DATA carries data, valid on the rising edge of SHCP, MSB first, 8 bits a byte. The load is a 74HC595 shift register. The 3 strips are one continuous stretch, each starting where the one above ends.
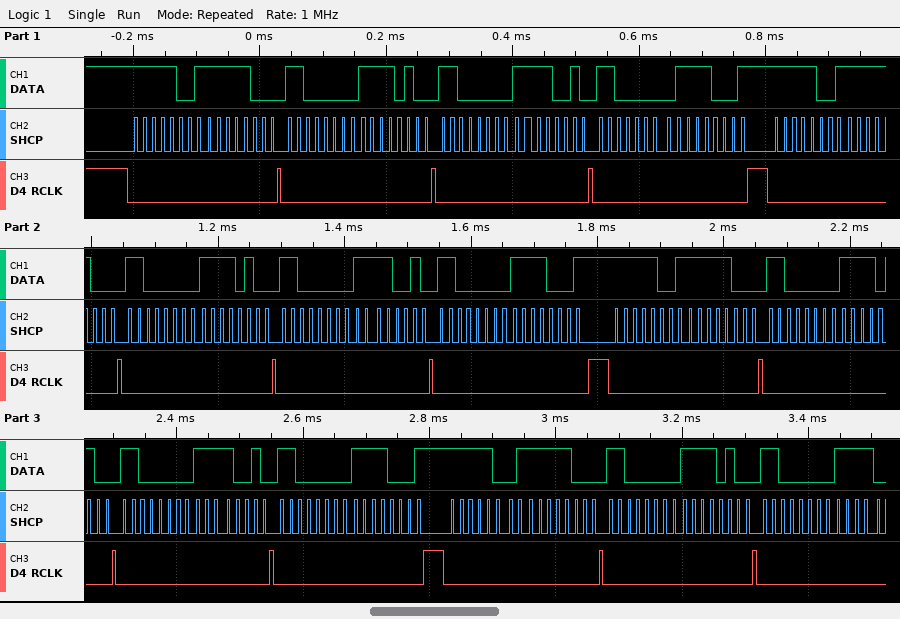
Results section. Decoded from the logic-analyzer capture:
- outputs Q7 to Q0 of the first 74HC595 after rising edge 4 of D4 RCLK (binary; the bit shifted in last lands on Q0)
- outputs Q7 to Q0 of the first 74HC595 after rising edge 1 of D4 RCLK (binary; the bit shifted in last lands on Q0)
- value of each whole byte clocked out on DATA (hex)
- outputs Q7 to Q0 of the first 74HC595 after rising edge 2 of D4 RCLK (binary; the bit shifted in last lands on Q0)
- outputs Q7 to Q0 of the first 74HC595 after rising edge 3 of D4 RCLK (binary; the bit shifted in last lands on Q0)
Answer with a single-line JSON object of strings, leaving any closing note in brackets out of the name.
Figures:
{"outputs Q7 to Q0 of the first 74HC595 after rising edge 4 of D4 RCLK": "11110001", "outputs Q7 to Q0 of the first 74HC595 after rising edge 1 of D4 RCLK": "11111000", "value of each whole byte clocked out on DATA": "F9 F8 C0 F4 C0 F2 C0 F1 F9 F8 C0 F4 C0 F2 C0 F1 F9 F8 C0 F4 C0 F2 C0 F1 F9 F8 C0 F4 C0", "outputs Q7 to Q0 of the first 74HC595 after rising edge 2 of D4 RCLK": "11110100", "outputs Q7 to Q0 of the first 74HC595 after rising edge 3 of D4 RCLK": "11110010"}
